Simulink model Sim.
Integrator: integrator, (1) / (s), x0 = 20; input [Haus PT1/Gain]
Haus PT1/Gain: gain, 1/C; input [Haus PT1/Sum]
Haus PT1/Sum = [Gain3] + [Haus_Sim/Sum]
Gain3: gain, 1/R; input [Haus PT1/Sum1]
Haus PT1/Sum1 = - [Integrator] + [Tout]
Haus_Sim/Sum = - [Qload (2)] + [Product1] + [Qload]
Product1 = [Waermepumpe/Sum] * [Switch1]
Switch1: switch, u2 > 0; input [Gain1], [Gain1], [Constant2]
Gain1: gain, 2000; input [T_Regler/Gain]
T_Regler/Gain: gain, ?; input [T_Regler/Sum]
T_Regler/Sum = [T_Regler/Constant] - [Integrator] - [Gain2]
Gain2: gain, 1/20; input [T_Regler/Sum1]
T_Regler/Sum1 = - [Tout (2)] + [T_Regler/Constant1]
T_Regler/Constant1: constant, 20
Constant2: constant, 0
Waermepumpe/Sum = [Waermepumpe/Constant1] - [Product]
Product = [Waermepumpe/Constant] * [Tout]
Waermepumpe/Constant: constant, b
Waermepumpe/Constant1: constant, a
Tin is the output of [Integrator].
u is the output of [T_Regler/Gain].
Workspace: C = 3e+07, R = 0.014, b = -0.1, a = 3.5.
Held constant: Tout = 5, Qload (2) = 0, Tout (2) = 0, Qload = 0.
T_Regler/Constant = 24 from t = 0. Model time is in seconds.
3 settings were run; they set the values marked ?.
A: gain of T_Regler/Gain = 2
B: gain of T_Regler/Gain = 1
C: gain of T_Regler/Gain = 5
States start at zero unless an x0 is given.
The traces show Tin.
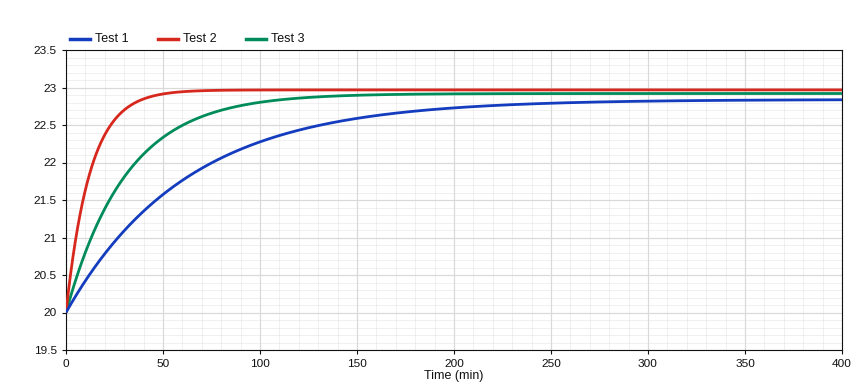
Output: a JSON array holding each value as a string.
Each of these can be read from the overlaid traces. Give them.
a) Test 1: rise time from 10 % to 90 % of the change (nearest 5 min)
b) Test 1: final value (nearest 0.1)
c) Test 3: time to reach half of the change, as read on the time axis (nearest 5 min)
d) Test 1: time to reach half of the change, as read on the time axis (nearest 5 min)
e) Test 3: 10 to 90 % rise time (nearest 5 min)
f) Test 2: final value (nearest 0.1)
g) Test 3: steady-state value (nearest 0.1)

["135 min", "22.8", "20 min", "45 min", "70 min", "23.0", "22.9"]
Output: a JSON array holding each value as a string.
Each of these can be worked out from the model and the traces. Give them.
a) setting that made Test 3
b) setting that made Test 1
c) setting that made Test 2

["A", "B", "C"]
